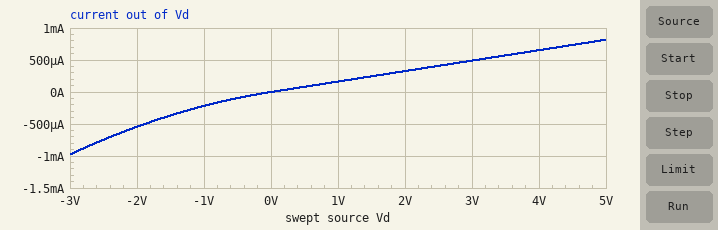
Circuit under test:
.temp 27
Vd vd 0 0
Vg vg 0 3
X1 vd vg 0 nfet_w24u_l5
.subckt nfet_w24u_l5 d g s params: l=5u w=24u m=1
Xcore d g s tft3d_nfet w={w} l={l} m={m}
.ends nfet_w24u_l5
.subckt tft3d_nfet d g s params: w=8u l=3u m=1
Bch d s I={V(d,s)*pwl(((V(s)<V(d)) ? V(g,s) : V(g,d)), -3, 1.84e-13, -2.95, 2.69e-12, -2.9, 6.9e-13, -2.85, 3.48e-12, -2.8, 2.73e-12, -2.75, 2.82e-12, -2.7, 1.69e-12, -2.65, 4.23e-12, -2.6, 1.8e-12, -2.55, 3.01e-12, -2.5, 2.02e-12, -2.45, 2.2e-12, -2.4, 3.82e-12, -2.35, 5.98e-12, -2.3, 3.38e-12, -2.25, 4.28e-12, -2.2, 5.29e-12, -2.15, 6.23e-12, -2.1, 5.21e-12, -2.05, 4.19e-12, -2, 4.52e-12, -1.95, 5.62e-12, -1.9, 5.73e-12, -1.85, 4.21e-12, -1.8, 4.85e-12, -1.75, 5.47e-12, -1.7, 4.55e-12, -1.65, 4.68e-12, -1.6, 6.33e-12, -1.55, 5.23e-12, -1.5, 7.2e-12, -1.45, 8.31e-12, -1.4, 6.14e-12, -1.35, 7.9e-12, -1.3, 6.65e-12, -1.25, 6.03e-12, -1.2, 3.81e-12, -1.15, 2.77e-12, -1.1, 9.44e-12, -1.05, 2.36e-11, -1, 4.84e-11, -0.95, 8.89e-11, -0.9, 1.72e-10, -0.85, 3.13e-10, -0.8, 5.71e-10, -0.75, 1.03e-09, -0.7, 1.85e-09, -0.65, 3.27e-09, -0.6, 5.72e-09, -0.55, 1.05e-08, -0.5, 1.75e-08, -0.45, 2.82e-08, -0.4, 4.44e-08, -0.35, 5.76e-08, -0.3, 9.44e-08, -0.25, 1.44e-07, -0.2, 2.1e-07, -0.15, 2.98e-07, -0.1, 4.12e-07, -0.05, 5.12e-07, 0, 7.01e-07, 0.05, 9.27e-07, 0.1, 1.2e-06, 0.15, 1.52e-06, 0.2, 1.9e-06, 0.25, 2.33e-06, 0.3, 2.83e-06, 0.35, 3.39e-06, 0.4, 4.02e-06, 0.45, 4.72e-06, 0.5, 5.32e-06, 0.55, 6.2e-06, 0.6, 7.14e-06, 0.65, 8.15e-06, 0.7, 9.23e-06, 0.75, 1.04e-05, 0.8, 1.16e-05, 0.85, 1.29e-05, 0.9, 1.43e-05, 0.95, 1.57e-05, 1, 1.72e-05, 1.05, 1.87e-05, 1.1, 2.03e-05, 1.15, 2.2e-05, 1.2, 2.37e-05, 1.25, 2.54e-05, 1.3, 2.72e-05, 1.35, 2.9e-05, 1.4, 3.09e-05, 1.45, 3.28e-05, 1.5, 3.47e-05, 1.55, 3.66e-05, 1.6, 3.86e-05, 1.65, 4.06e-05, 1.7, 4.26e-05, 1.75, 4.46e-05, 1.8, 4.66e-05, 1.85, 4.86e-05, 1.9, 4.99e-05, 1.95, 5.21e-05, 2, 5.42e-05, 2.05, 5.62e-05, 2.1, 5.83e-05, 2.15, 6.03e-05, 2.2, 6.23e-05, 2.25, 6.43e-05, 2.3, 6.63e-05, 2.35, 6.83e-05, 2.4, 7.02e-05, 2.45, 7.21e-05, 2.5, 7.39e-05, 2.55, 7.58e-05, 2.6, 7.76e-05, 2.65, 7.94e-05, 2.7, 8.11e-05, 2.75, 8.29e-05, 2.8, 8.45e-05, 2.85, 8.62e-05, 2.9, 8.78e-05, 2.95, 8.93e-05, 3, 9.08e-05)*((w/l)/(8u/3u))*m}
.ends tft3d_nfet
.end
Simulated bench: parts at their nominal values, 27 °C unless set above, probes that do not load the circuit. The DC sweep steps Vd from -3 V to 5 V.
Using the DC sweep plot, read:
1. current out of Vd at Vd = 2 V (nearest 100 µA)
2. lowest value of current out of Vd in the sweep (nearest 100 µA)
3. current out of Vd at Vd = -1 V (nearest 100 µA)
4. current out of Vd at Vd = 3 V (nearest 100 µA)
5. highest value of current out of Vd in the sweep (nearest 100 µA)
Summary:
300 µA
-1.0 mA
-200 µA
500 µA
800 µA
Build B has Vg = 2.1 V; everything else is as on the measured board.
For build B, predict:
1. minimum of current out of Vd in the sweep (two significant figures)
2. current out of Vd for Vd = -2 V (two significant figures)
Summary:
-830 µA
-450 µA
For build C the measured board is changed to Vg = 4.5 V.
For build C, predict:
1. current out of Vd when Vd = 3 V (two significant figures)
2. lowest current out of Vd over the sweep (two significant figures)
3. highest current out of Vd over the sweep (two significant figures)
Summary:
730 µA
-1.2 mA
1.2 mA
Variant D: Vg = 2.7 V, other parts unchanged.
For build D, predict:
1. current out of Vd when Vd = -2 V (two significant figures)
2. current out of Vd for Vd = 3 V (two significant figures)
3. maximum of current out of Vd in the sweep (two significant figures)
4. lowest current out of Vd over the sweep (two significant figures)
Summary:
-510 µA
440 µA
730 µA
-930 µA
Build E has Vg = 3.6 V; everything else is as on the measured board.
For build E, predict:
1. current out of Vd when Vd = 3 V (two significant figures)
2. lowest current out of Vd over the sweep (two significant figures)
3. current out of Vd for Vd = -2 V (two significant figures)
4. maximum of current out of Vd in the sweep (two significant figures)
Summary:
590 µA
-1.1 mA
-610 µA
980 µA
